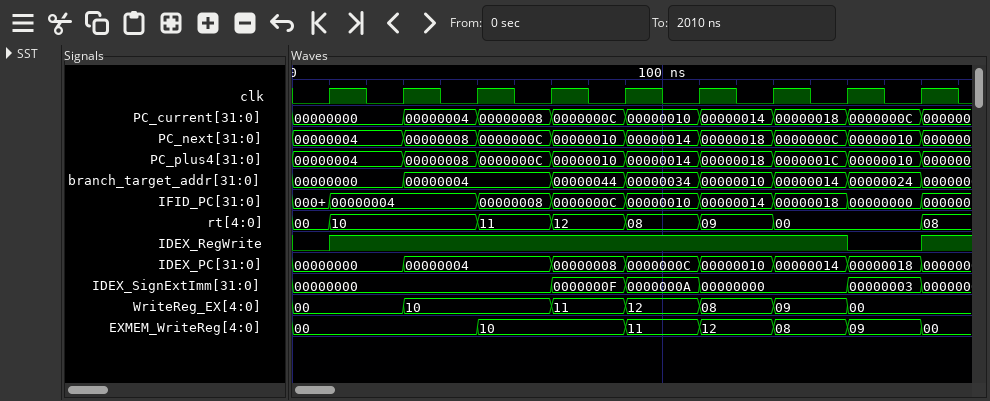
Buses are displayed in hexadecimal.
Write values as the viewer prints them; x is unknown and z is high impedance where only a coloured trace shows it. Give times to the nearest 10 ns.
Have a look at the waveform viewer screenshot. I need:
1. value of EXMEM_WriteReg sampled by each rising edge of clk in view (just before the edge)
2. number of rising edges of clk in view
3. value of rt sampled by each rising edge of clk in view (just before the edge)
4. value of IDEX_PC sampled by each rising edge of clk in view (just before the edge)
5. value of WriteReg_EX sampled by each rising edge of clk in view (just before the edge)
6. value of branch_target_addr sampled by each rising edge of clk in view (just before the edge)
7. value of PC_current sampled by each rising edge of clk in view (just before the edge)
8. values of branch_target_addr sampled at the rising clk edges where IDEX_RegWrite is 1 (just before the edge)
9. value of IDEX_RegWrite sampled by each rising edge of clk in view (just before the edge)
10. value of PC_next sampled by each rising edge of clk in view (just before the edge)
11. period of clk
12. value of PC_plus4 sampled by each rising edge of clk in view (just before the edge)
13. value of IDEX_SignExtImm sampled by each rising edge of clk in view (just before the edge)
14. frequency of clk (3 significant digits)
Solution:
00, 00, 00, 10, 10, 11, 12, 08, 09
9
00, 10, 10, 11, 12, 08, 09, 00, 00
00000000, 00000000, 00000004, 00000004, 00000008, 0000000C, 00000010, 00000014, 00000018
00, 00, 10, 10, 11, 12, 08, 09, 00
00000000, 00000000, 00000004, 00000004, 00000044, 00000034, 00000010, 00000014, 00000024
00000000, 00000000, 00000004, 00000008, 0000000C, 00000010, 00000014, 00000018, 0000000C
00000000, 00000004, 00000004, 00000044, 00000034, 00000010, 00000014
0 1 1 1 1 1 1 1 0
00000004, 00000004, 00000008, 0000000C, 00000010, 00000014, 00000018, 0000000C, 00000010
20 ns
00000004, 00000004, 00000008, 0000000C, 00000010, 00000014, 00000018, 0000001C, 00000010
00000000, 00000000, 00000000, 00000000, 0000000F, 0000000A, 00000000, 00000000, 00000003
50.0 MHz
